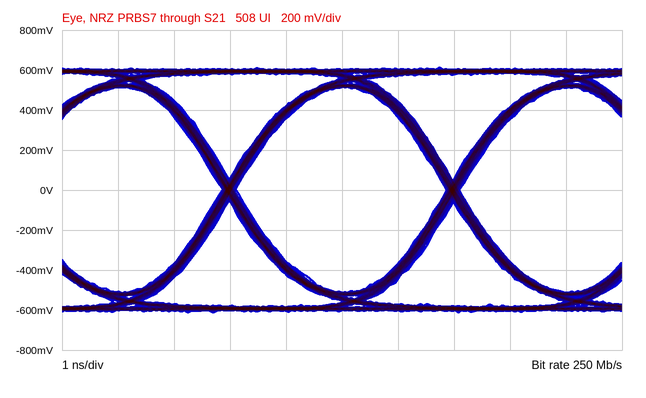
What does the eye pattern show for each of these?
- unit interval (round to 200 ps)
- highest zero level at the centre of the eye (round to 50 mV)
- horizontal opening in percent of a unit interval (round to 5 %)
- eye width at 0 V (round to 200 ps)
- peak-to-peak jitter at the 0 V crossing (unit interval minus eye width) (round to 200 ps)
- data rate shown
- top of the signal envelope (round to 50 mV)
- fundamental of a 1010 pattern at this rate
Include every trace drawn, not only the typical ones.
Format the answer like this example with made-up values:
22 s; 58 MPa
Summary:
4.0 ns; -500 mV; 95 %; 3.8 ns; 200 ps; 250 Mb/s; 600 mV; 125 MHz
